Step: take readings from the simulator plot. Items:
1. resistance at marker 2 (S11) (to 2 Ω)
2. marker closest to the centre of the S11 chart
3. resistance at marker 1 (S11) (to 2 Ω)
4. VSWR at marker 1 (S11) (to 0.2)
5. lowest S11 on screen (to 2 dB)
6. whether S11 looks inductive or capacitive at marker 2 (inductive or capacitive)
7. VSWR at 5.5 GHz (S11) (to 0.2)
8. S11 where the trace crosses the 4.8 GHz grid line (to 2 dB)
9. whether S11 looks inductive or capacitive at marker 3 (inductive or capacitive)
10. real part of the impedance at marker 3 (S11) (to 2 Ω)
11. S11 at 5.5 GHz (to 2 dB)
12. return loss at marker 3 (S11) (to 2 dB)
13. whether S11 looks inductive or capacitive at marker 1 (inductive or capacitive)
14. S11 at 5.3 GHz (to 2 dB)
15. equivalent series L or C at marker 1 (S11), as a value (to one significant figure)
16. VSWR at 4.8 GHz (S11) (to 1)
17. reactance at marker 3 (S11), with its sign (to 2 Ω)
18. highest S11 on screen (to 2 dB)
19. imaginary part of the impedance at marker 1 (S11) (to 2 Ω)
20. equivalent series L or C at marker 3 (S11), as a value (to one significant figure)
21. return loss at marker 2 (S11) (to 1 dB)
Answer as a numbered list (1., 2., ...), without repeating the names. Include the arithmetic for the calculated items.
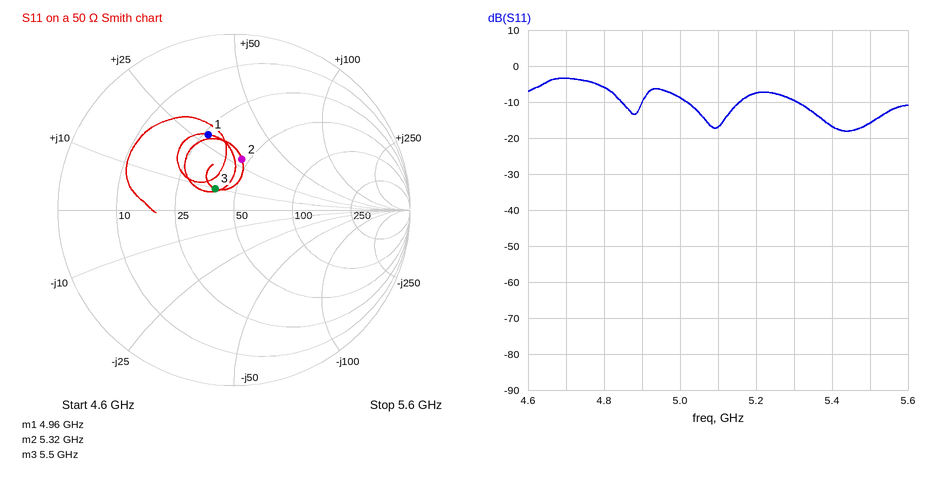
1. 46 Ω
2. marker 3
3. 26 Ω
4. 2.6
5. -18 dB
6. inductive
7. |Γ| = 10^(-16/20) = 0.1585; VSWR = (1 + 0.1585)/(1 − 0.1585) ≈ 1.4
8. -6 dB
9. inductive
10. 40 Ω
11. -16 dB
12. 16 dB
13. inductive
14. -10 dB
15. L = 28 Ω/(2π × 4.96 GHz) ≈ 898 pH, so 900 pH to one significant figure
16. |Γ| = 10^(-6/20) = 0.5012; VSWR = (1 + 0.5012)/(1 − 0.5012) ≈ 3
17. +10 Ω
18. -4 dB
19. +28 Ω
20. L = 10 Ω/(2π × 5.5 GHz) ≈ 289 pH, so 300 pH to one significant figure
21. 11 dB
